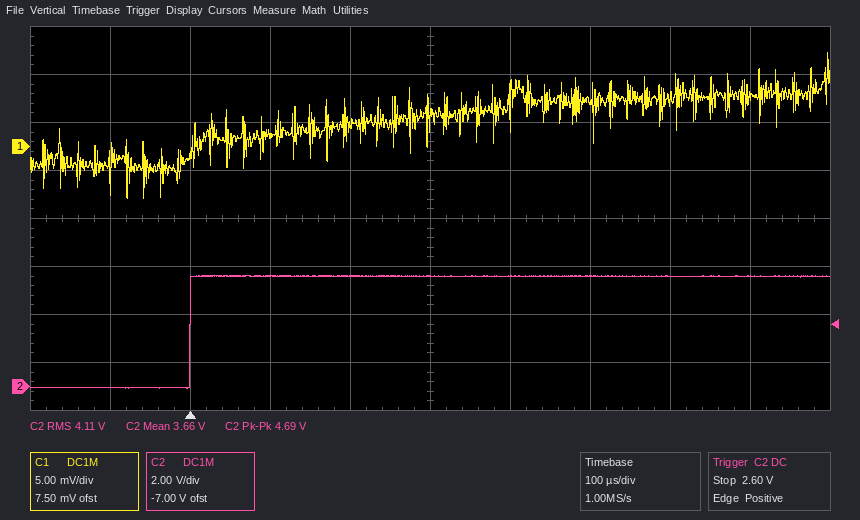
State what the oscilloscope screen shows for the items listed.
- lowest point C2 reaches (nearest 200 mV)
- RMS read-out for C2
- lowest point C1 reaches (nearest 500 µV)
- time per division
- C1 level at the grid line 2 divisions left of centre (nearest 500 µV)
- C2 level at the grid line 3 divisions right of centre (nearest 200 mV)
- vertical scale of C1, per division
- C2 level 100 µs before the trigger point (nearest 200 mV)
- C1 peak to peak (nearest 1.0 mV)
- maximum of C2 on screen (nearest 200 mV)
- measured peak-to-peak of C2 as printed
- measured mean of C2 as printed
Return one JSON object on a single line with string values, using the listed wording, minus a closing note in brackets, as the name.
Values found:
{"lowest point C2 reaches": "0.0 V", "RMS read-out for C2": "4.11 V", "lowest point C1 reaches": "-5.5 mV", "time per division": "100 µs", "C1 level at the grid line 2 divisions left of centre": "1.5 mV", "C2 level at the grid line 3 divisions right of centre": "4.6 V", "vertical scale of C1, per division": "5 mV", "C2 level 100 µs before the trigger point": "0.0 V", "C1 peak to peak": "15.0 mV", "maximum of C2 on screen": "4.6 V", "measured peak-to-peak of C2 as printed": "4.69 V", "measured mean of C2 as printed": "3.66 V"}
